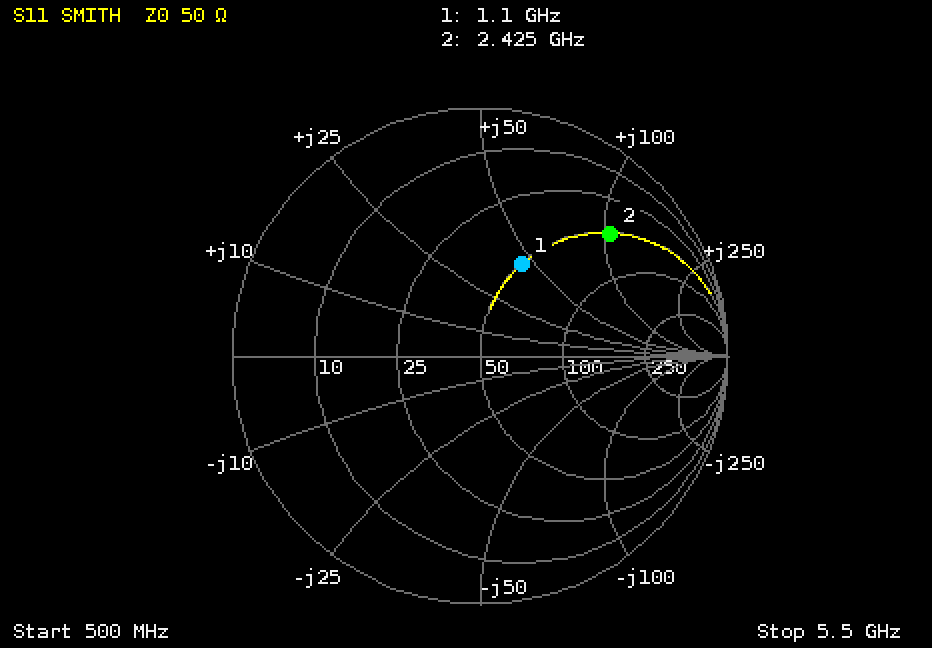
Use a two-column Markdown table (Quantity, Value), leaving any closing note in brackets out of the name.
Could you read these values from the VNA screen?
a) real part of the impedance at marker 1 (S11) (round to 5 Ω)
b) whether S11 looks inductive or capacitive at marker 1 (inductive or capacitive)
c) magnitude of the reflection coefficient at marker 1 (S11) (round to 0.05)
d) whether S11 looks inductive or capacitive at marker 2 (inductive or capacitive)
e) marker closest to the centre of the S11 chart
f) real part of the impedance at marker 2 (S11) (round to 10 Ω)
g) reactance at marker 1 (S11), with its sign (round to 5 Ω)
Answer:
| Quantity | Value |
|---|---|
| real part of the impedance at marker 1 (S11) | 50 Ω |
| whether S11 looks inductive or capacitive at marker 1 | inductive |
| magnitude of the reflection coefficient at marker 1 (S11) | 0.40 |
| whether S11 looks inductive or capacitive at marker 2 | inductive |
| marker closest to the centre of the S11 chart | marker 1 |
| real part of the impedance at marker 2 (S11) | 50 Ω |
| reactance at marker 1 (S11), with its sign | +45 Ω |
